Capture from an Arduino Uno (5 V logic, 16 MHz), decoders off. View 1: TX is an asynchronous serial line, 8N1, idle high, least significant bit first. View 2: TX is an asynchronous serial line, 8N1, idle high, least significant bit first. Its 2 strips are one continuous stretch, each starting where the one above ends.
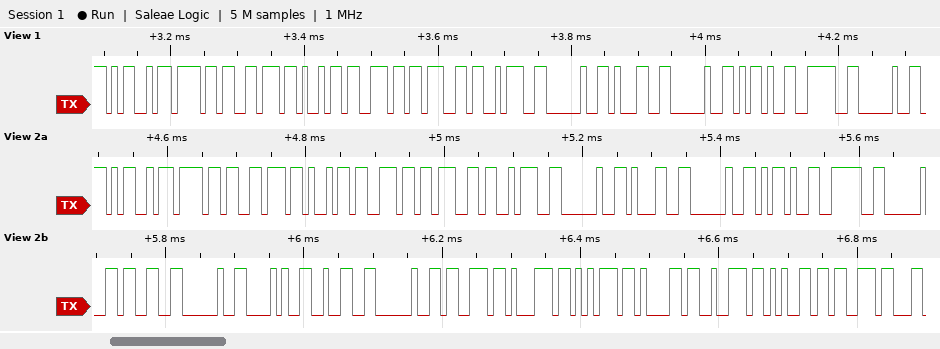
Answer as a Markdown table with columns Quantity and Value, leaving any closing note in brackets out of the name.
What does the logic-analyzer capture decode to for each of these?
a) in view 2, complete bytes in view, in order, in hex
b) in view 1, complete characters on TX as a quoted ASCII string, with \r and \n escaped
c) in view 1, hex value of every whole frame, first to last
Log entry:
| Quantity | Value |
|---|---|
| in view 2, complete bytes in view, in order, in hex | 4D 6F 76 69 6E 67 3A 20 31 20 2D 3E 20 33 20 28 32 20 73 71 75 61 72 65 73 |
| in view 1, complete characters on TX as a quoted ASCII string, with \r and \n escaped | "Moving: 1 -> " |
| in view 1, hex value of every whole frame, first to last | 4D 6F 76 69 6E 67 3A 20 31 20 2D 3E 20 |
